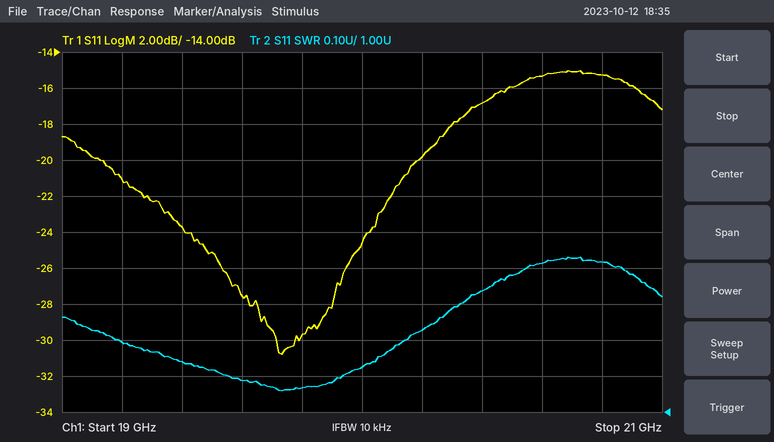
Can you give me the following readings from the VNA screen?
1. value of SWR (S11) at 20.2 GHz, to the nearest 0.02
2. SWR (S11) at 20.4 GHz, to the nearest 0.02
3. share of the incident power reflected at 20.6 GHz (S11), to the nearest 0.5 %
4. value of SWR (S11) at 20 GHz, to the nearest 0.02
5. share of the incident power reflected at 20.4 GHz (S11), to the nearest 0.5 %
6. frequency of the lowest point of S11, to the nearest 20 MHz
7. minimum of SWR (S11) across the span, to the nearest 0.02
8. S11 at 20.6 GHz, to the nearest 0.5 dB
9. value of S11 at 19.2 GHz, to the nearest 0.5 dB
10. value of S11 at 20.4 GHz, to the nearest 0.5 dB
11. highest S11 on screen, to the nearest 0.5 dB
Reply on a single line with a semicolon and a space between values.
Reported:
1.22; 1.34; 3.0 %; 1.12; 2.0 %; 19.74 GHz; 1.06; -15.5 dB; -21.0 dB; -17.0 dB; -15.0 dB
